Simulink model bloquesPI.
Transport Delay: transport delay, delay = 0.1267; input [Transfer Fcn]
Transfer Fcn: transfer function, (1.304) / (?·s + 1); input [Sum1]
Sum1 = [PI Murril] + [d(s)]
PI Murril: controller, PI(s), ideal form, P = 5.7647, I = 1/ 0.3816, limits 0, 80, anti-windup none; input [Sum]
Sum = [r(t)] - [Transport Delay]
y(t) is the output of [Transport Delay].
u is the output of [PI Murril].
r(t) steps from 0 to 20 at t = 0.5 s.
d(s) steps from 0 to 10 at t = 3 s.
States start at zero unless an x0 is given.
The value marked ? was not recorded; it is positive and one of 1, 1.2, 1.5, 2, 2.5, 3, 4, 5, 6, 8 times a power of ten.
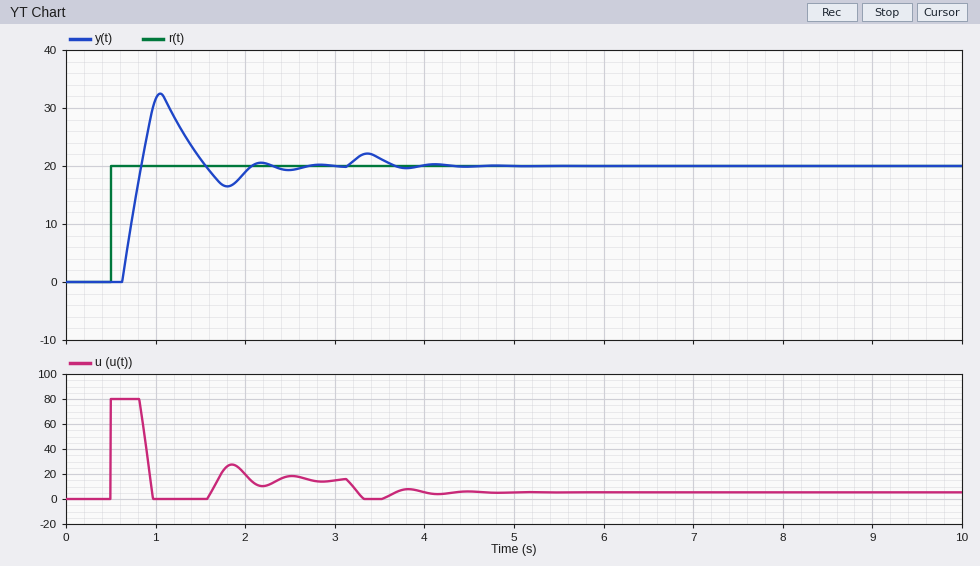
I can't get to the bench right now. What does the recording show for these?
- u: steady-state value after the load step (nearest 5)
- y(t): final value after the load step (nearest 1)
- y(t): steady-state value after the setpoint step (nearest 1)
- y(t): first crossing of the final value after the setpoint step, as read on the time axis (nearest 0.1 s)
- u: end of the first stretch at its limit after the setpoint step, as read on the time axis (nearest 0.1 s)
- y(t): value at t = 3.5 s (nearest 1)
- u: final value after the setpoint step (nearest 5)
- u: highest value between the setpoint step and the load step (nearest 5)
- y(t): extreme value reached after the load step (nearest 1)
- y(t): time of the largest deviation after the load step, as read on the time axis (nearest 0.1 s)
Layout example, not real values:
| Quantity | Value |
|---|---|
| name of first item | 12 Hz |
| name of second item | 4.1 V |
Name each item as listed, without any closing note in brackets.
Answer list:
| Quantity | Value |
|---|---|
| u: steady-state value after the load step | 5 |
| y(t): final value after the load step | 20 |
| y(t): steady-state value after the setpoint step | 20 |
| y(t): first crossing of the final value after the setpoint step, as read on the time axis | 0.8 s |
| u: end of the first stretch at its limit after the setpoint step, as read on the time axis | 0.8 s |
| y(t): value at t = 3.5 s | 21 |
| u: final value after the setpoint step | 15 |
| u: highest value between the setpoint step and the load step | 80 |
| y(t): extreme value reached after the load step | 22 |
| y(t): time of the largest deviation after the load step, as read on the time axis | 3.4 s |
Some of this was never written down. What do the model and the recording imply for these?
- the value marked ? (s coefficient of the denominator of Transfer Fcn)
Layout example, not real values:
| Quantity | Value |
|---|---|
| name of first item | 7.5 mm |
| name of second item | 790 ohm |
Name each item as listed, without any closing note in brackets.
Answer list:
| Quantity | Value |
|---|---|
| the value marked ? | 1 |
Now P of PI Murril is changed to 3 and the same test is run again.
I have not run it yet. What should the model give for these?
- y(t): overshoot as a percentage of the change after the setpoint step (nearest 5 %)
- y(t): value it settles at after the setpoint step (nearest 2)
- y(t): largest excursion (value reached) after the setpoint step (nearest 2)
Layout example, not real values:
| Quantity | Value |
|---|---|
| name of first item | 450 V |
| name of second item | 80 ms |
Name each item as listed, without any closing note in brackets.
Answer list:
| Quantity | Value |
|---|---|
| y(t): overshoot as a percentage of the change after the setpoint step | 35 % |
| y(t): value it settles at after the setpoint step | 20 |
| y(t): largest excursion (value reached) after the setpoint step | 26 |
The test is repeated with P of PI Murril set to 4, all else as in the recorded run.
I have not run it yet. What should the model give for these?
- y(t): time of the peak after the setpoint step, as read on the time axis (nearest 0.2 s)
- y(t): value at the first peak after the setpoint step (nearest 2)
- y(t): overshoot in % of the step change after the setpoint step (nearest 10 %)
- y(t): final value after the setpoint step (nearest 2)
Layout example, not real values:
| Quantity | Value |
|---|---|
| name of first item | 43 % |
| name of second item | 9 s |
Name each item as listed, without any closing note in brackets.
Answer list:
| Quantity | Value |
|---|---|
| y(t): time of the peak after the setpoint step, as read on the time axis | 1.0 s |
| y(t): value at the first peak after the setpoint step | 30 |
| y(t): overshoot in % of the step change after the setpoint step | 50 % |
| y(t): final value after the setpoint step | 20 |
